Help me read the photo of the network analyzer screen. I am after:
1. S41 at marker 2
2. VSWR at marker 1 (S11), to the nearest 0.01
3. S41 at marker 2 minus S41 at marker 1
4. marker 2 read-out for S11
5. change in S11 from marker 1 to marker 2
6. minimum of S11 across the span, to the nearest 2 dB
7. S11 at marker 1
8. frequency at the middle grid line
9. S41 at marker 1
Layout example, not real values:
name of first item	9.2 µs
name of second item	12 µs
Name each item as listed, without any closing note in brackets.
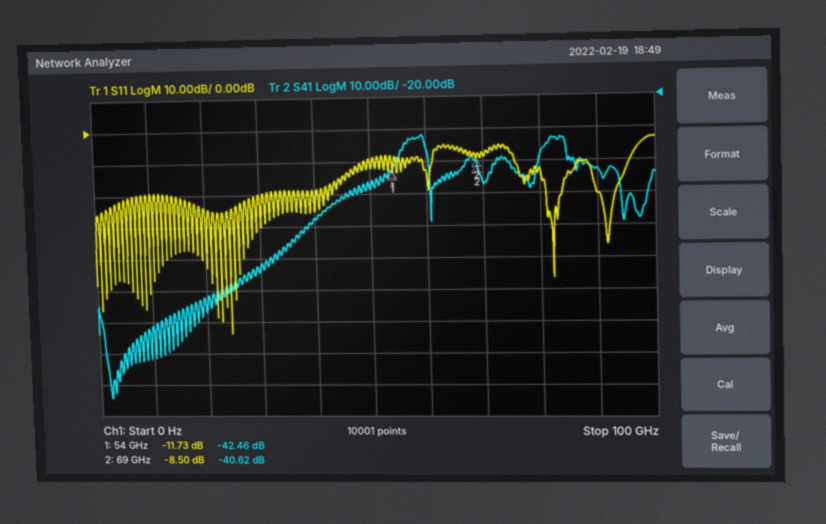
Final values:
S41 at marker 2	-40.62 dB
VSWR at marker 1 (S11), to the nearest 0.01	1.70
S41 at marker 2 minus S41 at marker 1	1.84 dB
marker 2 read-out for S11	-8.50 dB
change in S11 from marker 1 to marker 2	3.23 dB
minimum of S11 across the span, to the nearest 2 dB	-64 dB
S11 at marker 1	-11.73 dB
frequency at the middle grid line	50 GHz
S41 at marker 1	-42.46 dB
